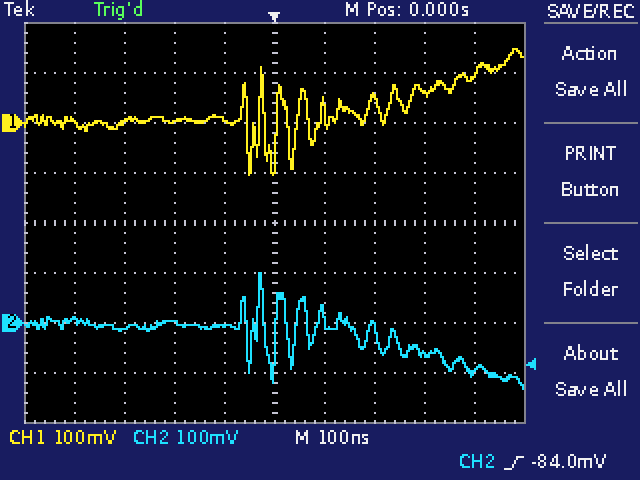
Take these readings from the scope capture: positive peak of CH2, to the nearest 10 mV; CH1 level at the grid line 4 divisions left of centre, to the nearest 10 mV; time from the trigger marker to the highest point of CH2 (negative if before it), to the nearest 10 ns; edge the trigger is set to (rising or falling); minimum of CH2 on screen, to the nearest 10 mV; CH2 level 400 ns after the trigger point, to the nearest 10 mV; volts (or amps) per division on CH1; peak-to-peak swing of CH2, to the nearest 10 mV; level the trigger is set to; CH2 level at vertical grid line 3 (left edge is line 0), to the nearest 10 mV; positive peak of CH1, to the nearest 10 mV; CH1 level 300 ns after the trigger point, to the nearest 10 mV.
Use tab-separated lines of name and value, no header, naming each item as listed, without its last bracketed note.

positive peak of CH2, to the nearest 10 mV	100 mV
CH1 level at the grid line 4 divisions left of centre, to the nearest 10 mV	0 mV
time from the trigger marker to the highest point of CH2 (negative if before it), to the nearest 10 ns	-30 ns
edge the trigger is set to	rising
minimum of CH2 on screen, to the nearest 10 mV	-130 mV
CH2 level 400 ns after the trigger point, to the nearest 10 mV	-100 mV
volts (or amps) per division on CH1	100 mV
peak-to-peak swing of CH2, to the nearest 10 mV	230 mV
level the trigger is set to	-84.0 mV
CH2 level at vertical grid line 3 (left edge is line 0), to the nearest 10 mV	0 mV
positive peak of CH1, to the nearest 10 mV	150 mV
CH1 level 300 ns after the trigger point, to the nearest 10 mV	60 mV
